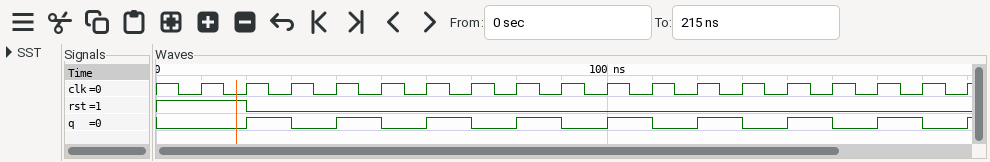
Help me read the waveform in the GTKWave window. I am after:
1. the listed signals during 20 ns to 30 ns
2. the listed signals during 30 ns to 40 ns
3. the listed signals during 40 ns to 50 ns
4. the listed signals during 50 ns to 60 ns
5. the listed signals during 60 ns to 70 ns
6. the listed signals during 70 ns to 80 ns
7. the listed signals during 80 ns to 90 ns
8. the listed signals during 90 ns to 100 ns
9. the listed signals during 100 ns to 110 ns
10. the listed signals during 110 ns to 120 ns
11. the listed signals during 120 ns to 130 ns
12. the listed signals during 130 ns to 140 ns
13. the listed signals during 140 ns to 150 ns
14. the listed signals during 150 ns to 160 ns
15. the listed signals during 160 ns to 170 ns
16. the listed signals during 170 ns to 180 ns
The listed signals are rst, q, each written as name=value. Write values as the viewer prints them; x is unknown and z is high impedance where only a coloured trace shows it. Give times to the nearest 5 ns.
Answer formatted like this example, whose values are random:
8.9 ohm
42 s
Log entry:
rst=0, q=1
rst=0, q=0
rst=0, q=1
rst=0, q=0
rst=0, q=1
rst=0, q=0
rst=0, q=1
rst=0, q=0
rst=0, q=1
rst=0, q=0
rst=0, q=1
rst=0, q=0
rst=0, q=1
rst=0, q=0
rst=0, q=1
rst=0, q=0
